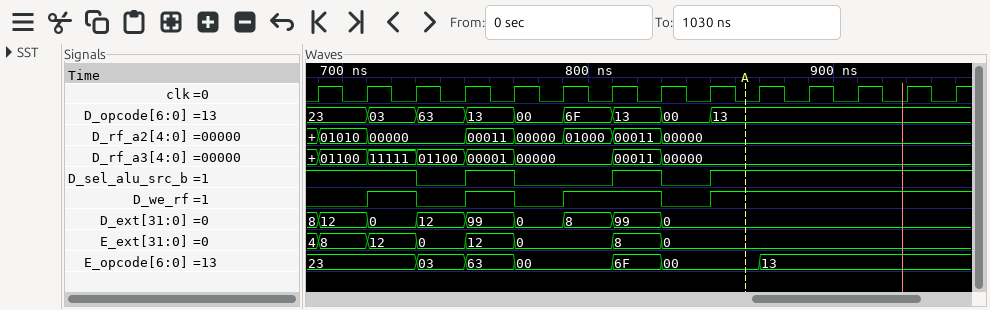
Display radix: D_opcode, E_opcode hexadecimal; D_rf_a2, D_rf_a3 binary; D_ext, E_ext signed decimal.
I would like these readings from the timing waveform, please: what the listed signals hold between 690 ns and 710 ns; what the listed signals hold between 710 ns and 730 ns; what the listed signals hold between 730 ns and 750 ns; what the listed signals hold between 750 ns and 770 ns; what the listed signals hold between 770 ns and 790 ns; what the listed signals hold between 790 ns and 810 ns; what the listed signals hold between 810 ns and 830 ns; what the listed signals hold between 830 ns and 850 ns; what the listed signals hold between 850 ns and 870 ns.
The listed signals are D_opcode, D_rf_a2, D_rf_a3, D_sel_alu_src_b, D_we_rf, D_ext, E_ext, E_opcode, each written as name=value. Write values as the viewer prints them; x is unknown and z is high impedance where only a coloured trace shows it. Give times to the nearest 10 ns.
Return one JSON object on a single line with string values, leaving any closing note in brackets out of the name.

{"what the listed signals hold between 690 ns and 710 ns": "D_opcode=23, D_rf_a2=01010, D_rf_a3=01100, D_sel_alu_src_b=1, D_we_rf=0, D_ext=12, E_ext=8, E_opcode=23", "what the listed signals hold between 710 ns and 730 ns": "D_opcode=03, D_rf_a2=00000, D_rf_a3=11111, D_sel_alu_src_b=1, D_we_rf=1, D_ext=0, E_ext=12, E_opcode=23", "what the listed signals hold between 730 ns and 750 ns": "D_opcode=63, D_rf_a2=00000, D_rf_a3=01100, D_sel_alu_src_b=0, D_we_rf=0, D_ext=12, E_ext=0, E_opcode=03", "what the listed signals hold between 750 ns and 770 ns": "D_opcode=13, D_rf_a2=00011, D_rf_a3=00001, D_sel_alu_src_b=1, D_we_rf=1, D_ext=99, E_ext=12, E_opcode=63", "what the listed signals hold between 770 ns and 790 ns": "D_opcode=00, D_rf_a2=00000, D_rf_a3=00000, D_sel_alu_src_b=0, D_we_rf=0, D_ext=0, E_ext=0, E_opcode=00", "what the listed signals hold between 790 ns and 810 ns": "D_opcode=6F, D_rf_a2=01000, D_rf_a3=00000, D_sel_alu_src_b=0, D_we_rf=1, D_ext=8, E_ext=0, E_opcode=00", "what the listed signals hold between 810 ns and 830 ns": "D_opcode=13, D_rf_a2=00011, D_rf_a3=00011, D_sel_alu_src_b=1, D_we_rf=1, D_ext=99, E_ext=8, E_opcode=6F", "what the listed signals hold between 830 ns and 850 ns": "D_opcode=00, D_rf_a2=00000, D_rf_a3=00000, D_sel_alu_src_b=0, D_we_rf=0, D_ext=0, E_ext=0, E_opcode=00", "what the listed signals hold between 850 ns and 870 ns": "D_opcode=13, D_rf_a2=00000, D_rf_a3=00000, D_sel_alu_src_b=1, D_we_rf=1, D_ext=0, E_ext=0, E_opcode=00"}
